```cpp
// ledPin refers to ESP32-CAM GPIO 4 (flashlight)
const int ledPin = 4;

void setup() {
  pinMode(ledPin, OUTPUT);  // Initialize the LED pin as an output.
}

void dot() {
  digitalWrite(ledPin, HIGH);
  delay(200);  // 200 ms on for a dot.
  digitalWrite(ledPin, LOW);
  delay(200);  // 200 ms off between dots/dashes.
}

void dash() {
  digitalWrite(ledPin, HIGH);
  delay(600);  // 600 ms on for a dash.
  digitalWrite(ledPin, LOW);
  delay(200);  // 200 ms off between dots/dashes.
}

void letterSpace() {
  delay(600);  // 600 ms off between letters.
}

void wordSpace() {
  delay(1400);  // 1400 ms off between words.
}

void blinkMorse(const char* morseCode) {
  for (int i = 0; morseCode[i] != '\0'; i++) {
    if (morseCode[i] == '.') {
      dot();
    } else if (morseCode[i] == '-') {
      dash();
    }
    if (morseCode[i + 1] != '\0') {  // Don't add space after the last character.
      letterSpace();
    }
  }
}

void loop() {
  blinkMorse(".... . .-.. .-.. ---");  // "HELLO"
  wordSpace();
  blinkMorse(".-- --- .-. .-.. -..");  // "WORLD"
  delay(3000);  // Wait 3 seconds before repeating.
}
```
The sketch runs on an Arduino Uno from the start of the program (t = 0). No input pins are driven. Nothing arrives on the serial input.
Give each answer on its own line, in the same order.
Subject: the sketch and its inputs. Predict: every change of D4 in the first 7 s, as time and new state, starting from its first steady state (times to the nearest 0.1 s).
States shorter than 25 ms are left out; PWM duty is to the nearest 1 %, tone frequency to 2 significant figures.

0 s high; 0.2 s low; 1 s high; 1.2 s low; 2 s high; 2.2 s low; 3 s high; 3.2 s low; 4.6 s high; 4.8 s low; 6.2 s high; 6.4 s low
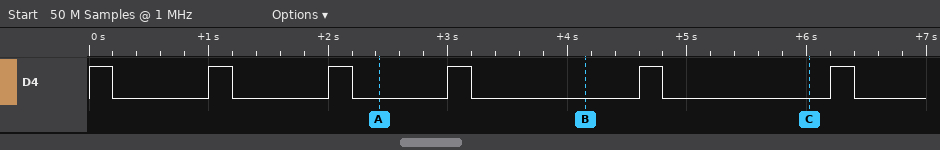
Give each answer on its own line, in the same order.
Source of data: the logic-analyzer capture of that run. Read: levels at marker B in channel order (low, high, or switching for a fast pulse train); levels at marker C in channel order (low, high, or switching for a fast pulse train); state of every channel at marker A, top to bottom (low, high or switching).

D4 low
D4 low
D4 low
